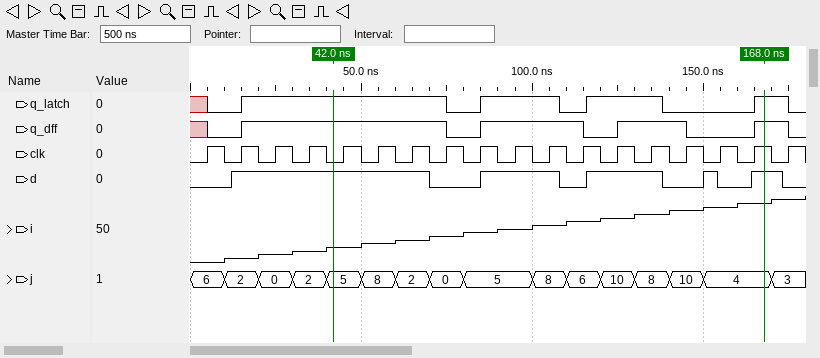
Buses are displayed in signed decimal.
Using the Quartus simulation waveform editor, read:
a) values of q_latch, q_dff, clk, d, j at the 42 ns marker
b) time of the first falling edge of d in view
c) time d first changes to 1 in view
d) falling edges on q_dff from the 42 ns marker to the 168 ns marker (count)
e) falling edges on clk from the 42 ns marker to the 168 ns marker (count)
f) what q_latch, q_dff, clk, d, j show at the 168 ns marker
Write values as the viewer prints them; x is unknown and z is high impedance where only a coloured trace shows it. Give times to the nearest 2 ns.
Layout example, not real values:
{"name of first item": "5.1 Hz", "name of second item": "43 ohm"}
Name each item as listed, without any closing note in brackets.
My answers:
{"values of q_latch, q_dff, clk, d, j at the 42 ns marker": "q_latch=1, q_dff=1, clk=0, d=1, j=5", "time of the first falling edge of d in view": "70 ns", "time d first changes to 1 in view": "12 ns", "falling edges on q_dff from the 42 ns marker to the 168 ns marker": "3", "falling edges on clk from the 42 ns marker to the 168 ns marker": "12", "what q_latch, q_dff, clk, d, j show at the 168 ns marker": "q_latch=1, q_dff=1, clk=1, d=1, j=4"}
